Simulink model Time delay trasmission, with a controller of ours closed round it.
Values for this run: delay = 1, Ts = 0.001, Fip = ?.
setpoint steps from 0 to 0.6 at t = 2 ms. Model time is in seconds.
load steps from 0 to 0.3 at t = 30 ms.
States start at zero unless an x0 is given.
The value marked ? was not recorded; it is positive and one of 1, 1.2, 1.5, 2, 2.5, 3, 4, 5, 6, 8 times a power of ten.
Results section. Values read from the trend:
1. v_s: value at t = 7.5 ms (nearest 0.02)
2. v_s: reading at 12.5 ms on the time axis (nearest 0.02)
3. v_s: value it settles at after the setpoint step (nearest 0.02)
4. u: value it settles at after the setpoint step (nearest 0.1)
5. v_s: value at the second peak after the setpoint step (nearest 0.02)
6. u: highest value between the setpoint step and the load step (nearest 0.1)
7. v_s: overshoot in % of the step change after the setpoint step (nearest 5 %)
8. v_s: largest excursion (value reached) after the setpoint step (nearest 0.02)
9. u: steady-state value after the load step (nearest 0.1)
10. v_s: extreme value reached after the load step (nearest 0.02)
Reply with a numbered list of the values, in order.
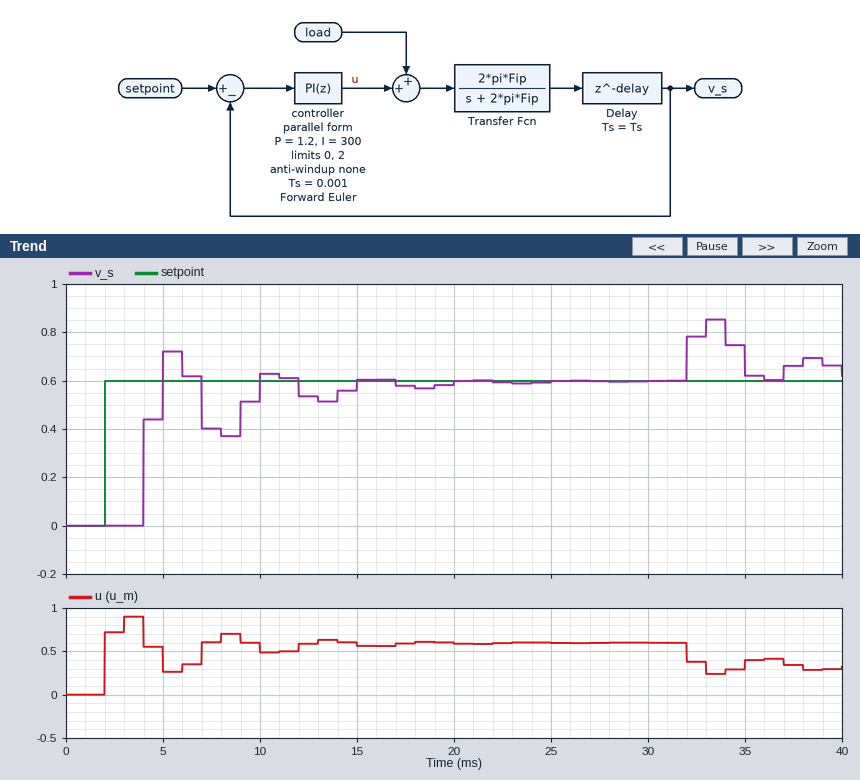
1. 0.40
2. 0.54
3. 0.60
4. 0.6
5. 0.62
6. 0.9
7. 20 %
8. 0.72
9. 0.3
10. 0.86
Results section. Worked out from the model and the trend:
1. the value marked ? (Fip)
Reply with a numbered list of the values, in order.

1. 150
